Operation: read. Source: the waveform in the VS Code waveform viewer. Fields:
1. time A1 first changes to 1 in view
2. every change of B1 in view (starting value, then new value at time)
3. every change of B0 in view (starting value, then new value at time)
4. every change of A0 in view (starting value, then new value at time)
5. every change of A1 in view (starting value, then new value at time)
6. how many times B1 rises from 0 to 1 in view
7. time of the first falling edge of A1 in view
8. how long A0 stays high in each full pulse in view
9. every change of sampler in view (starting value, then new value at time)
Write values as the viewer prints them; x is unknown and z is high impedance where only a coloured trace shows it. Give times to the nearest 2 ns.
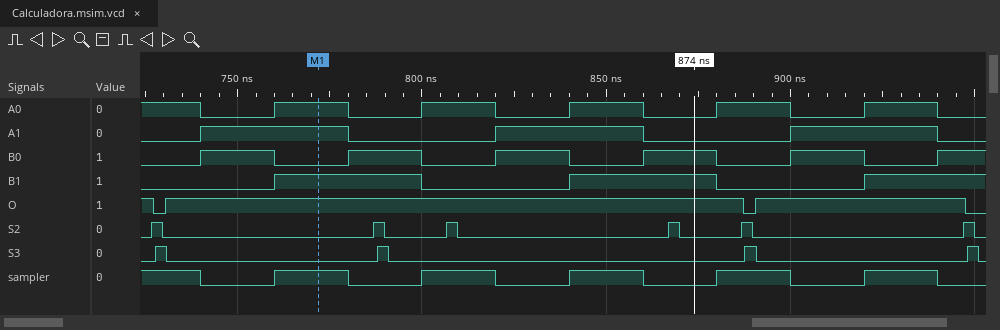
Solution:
740 ns
0, 1 at 760 ns, 0 at 800 ns, 1 at 840 ns, 0 at 880 ns, 1 at 920 ns
0, 1 at 740 ns, 0 at 760 ns, 1 at 780 ns, 0 at 800 ns, 1 at 820 ns, 0 at 840 ns, 1 at 860 ns, 0 at 880 ns, 1 at 900 ns, 0 at 920 ns, 1 at 940 ns
1, 0 at 740 ns, 1 at 760 ns, 0 at 780 ns, 1 at 800 ns, 0 at 820 ns, 1 at 840 ns, 0 at 860 ns, 1 at 880 ns, 0 at 900 ns, 1 at 920 ns, 0 at 940 ns
0, 1 at 740 ns, 0 at 780 ns, 1 at 820 ns, 0 at 860 ns, 1 at 900 ns, 0 at 940 ns
3
780 ns
20 ns, 20 ns, 20 ns, 20 ns, 20 ns
1, 0 at 740 ns, 1 at 760 ns, 0 at 780 ns, 1 at 800 ns, 0 at 820 ns, 1 at 840 ns, 0 at 860 ns, 1 at 880 ns, 0 at 900 ns, 1 at 920 ns, 0 at 940 ns
